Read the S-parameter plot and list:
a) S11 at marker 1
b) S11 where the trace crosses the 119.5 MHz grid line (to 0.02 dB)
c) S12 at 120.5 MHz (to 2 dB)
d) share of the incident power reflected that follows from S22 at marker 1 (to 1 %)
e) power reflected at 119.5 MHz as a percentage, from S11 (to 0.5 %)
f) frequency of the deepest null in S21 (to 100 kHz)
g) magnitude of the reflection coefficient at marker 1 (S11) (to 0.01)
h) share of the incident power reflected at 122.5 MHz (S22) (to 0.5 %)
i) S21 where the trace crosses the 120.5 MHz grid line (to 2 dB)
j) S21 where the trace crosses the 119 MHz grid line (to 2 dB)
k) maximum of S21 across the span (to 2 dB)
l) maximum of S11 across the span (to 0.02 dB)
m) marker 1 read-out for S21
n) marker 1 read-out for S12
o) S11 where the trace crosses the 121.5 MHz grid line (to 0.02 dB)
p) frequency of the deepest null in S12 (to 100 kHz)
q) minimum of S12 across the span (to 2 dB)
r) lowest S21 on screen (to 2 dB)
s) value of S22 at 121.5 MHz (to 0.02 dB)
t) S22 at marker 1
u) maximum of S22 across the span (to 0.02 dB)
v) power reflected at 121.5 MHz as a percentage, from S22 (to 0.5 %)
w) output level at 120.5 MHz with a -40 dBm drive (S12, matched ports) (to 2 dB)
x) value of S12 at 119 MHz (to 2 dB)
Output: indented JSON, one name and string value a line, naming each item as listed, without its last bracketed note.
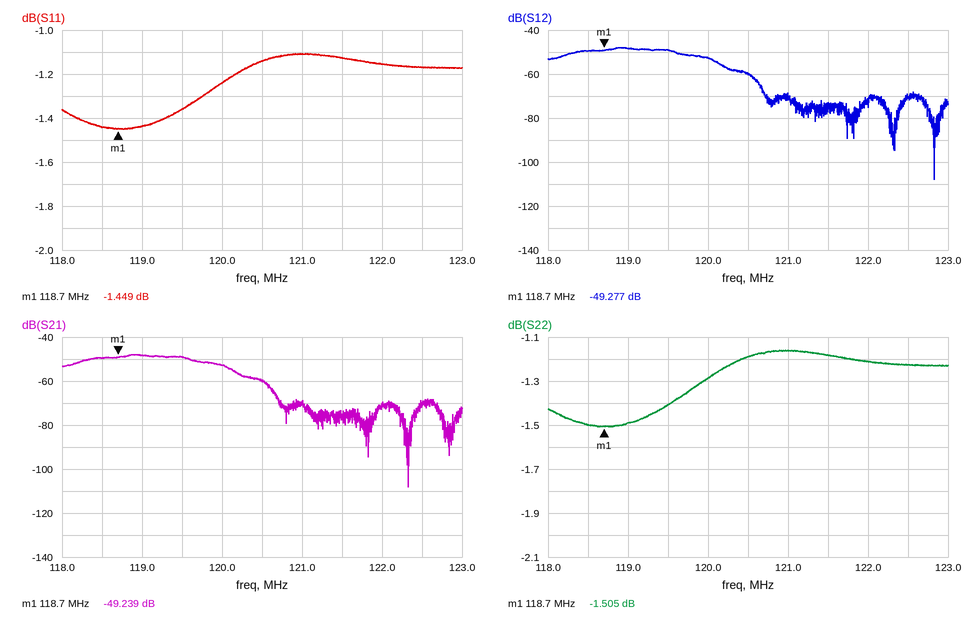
{
  "S11 at marker 1": "-1.449 dB",
  "S11 where the trace crosses the 119.5 MHz grid line": "-1.36 dB",
  "S12 at 120.5 MHz": "-60 dB",
  "share of the incident power reflected that follows from S22 at marker 1": "71 %",
  "power reflected at 119.5 MHz as a percentage, from S11": "73.0 %",
  "frequency of the deepest null in S21": "122.3 MHz",
  "magnitude of the reflection coefficient at marker 1 (S11)": "0.85",
  "share of the incident power reflected at 122.5 MHz (S22)": "75.5 %",
  "S21 where the trace crosses the 120.5 MHz grid line": "-60 dB",
  "S21 where the trace crosses the 119 MHz grid line": "-48 dB",
  "maximum of S21 across the span": "-48 dB",
  "maximum of S11 across the span": "-1.10 dB",
  "marker 1 read-out for S21": "-49.239 dB",
  "marker 1 read-out for S12": "-49.277 dB",
  "S11 where the trace crosses the 121.5 MHz grid line": "-1.12 dB",
  "frequency of the deepest null in S12": "122.8 MHz",
  "minimum of S12 across the span": "-108 dB",
  "lowest S21 on screen": "-108 dB",
  "value of S22 at 121.5 MHz": "-1.18 dB",
  "S22 at marker 1": "-1.505 dB",
  "maximum of S22 across the span": "-1.16 dB",
  "power reflected at 121.5 MHz as a percentage, from S22": "76.0 %",
  "output level at 120.5 MHz with a -40 dBm drive (S12, matched ports)": "-100 dBm",
  "value of S12 at 119 MHz": "-48 dB"
}
